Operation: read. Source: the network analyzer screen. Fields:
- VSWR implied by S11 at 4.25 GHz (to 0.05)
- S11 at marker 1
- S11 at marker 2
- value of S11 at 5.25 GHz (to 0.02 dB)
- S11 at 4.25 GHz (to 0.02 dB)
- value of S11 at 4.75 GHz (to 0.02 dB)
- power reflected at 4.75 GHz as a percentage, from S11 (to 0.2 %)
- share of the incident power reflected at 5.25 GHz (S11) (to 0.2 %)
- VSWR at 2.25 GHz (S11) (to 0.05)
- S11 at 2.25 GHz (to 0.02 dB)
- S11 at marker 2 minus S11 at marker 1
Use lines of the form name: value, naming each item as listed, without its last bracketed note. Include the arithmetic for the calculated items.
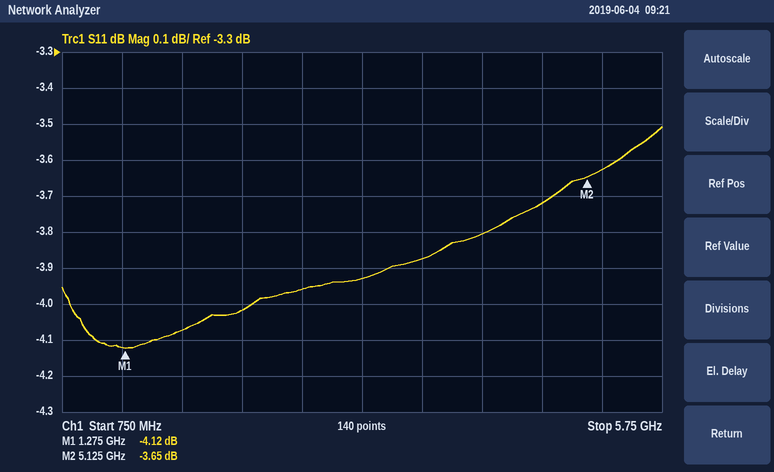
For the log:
VSWR implied by S11 at 4.25 GHz: |Γ| = 10^(-3.8/20) = 0.6457; VSWR = (1 + 0.6457)/(1 − 0.6457) ≈ 4.64, so 4.65 to the nearest 0.05
S11 at marker 1: -4.12 dB
S11 at marker 2: -3.65 dB
value of S11 at 5.25 GHz: -3.62 dB
S11 at 4.25 GHz: -3.80 dB
value of S11 at 4.75 GHz: -3.72 dB
power reflected at 4.75 GHz as a percentage, from S11: 10^(-3.72/10) ≈ 42.5 %, so 42.4 % to the nearest 0.2 %
share of the incident power reflected at 5.25 GHz (S11): 10^(-3.62/10) ≈ 43.5 %, so 43.4 % to the nearest 0.2 %
VSWR at 2.25 GHz (S11): |Γ| = 10^(-4.02/20) = 0.6295; VSWR = (1 + 0.6295)/(1 − 0.6295) ≈ 4.40
S11 at 2.25 GHz: -4.02 dB
S11 at marker 2 minus S11 at marker 1: -3.65 − (-4.12) = 0.47 dB
